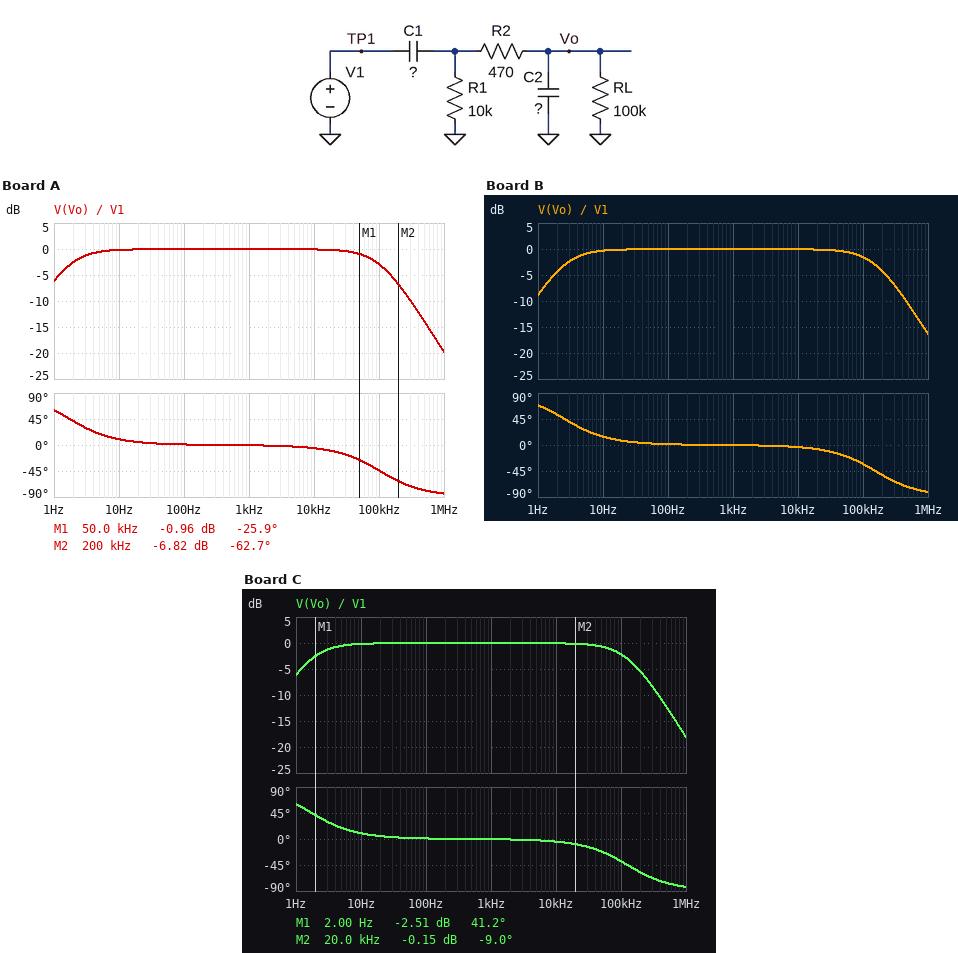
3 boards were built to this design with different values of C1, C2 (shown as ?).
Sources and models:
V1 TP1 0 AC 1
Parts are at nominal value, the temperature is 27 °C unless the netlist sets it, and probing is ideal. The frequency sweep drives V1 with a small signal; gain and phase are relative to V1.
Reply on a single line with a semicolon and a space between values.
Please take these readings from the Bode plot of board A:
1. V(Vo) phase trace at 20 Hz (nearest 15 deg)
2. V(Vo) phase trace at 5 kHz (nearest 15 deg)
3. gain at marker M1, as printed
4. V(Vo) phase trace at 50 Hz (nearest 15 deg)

0 deg; 0 deg; -0.96 dB; 0 deg
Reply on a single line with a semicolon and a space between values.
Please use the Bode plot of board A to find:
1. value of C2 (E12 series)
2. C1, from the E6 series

3.3 nF; 10 µF
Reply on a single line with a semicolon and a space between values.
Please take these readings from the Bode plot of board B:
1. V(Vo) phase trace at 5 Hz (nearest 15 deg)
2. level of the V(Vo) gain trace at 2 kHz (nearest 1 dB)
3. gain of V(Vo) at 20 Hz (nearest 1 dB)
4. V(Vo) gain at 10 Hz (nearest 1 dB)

30 deg; 0 dB; 0 dB; 0 dB
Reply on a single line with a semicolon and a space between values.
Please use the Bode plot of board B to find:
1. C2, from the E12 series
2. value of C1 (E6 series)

2.2 nF; 6.8 µF
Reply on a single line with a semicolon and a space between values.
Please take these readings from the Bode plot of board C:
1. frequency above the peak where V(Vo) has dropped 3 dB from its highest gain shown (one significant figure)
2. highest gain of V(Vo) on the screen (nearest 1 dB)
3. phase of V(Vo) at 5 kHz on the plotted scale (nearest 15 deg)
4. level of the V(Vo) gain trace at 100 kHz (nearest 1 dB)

100 kHz; 0 dB; 0 deg; -2 dB
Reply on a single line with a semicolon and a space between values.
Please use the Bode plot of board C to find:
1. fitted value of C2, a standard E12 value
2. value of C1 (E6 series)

2.7 nF; 10 µF
